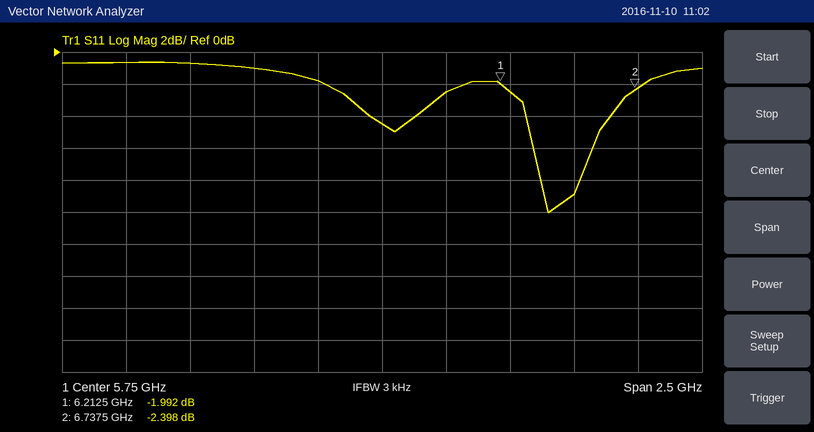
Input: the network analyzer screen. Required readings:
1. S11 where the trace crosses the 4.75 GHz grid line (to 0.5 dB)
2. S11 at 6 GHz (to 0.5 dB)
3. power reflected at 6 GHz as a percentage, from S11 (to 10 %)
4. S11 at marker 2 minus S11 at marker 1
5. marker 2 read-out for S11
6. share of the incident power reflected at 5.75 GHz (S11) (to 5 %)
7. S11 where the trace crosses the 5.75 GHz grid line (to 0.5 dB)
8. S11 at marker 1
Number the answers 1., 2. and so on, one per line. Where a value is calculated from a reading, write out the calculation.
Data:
1. -0.5 dB
2. -2.5 dB
3. 10^(-2.5/10) ≈ 56.2 %, so 60 % to the nearest 10 %
4. -2.398 − (-1.992) = -0.406 dB
5. -2.398 dB
6. 10^(-4.5/10) ≈ 35 %
7. -4.5 dB
8. -1.992 dB
